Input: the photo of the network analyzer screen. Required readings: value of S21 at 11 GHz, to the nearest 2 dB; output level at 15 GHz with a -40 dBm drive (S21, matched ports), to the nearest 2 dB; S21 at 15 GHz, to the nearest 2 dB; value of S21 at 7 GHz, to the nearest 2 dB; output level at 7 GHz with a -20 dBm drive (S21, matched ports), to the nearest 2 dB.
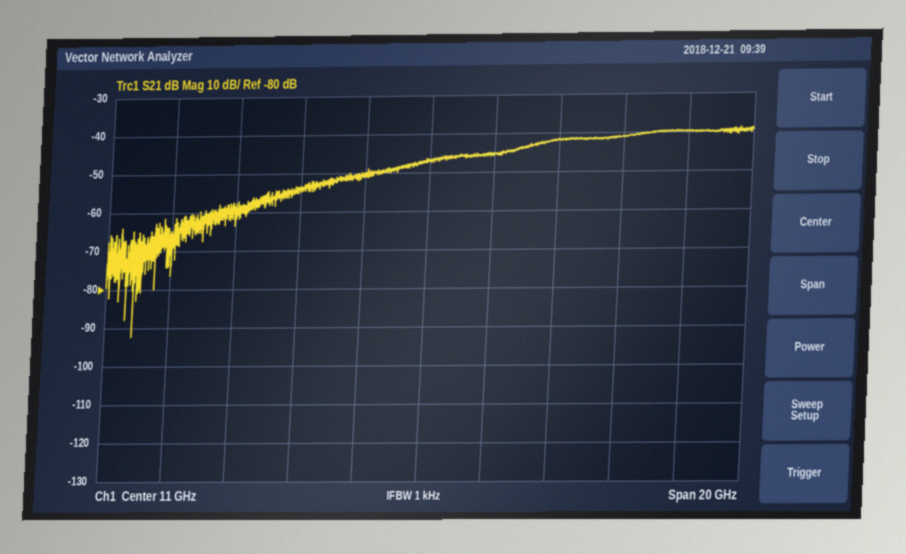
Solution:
-46 dB
-82 dBm
-42 dB
-54 dB
-74 dBm
